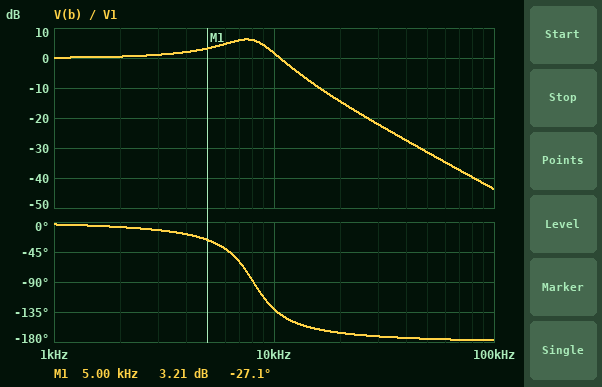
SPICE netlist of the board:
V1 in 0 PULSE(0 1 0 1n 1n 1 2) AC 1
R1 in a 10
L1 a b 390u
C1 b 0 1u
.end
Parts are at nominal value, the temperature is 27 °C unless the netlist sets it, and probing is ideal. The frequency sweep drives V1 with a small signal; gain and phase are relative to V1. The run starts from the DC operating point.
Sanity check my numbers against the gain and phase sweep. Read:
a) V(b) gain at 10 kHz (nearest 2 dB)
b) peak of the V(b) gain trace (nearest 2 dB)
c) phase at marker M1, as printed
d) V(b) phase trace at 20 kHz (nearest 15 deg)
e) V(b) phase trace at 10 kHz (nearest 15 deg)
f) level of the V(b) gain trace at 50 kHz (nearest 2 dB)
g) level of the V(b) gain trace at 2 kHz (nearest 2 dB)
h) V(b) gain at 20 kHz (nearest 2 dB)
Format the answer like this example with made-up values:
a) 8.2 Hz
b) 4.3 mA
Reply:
a) 2 dB
b) 6 dB
c) -27.1 deg
d) -165 deg
e) -135 deg
f) -32 dB
g) 0 dB
h) -14 dB
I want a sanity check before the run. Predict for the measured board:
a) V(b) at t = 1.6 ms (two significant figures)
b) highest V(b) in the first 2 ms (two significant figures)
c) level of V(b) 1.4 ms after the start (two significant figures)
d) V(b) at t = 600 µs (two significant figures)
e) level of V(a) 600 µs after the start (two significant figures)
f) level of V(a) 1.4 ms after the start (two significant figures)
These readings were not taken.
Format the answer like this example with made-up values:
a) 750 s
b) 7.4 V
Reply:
a) 1.0 V
b) 1.4 V
c) 1.0 V
d) 1.0 V
e) 1.0 V
f) 1.0 V
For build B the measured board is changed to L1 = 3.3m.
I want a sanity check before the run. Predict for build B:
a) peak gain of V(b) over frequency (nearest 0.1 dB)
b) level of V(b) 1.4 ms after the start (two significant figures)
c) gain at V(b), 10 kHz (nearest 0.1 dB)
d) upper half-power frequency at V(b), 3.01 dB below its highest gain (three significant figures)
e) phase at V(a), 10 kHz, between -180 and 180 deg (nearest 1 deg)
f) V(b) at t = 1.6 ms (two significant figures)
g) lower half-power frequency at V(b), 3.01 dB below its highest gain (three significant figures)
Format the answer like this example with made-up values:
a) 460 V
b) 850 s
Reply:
a) 15.2 dB
b) 930 mV
c) -21.6 dB
d) 2.98 kHz
e) 3 deg
f) 1.1 V
g) 2.50 kHz
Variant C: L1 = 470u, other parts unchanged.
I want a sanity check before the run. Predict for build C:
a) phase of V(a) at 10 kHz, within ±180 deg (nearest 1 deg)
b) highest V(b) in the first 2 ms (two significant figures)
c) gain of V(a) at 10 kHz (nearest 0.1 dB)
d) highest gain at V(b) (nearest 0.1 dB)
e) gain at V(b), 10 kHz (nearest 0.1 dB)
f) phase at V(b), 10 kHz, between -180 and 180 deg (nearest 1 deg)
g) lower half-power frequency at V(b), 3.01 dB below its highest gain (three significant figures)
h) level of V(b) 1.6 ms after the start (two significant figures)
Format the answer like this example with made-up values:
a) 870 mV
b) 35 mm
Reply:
a) 36 deg
b) 1.5 V
c) -1.9 dB
d) 7.0 dB
e) -0.5 dB
f) -144 deg
g) 4.90 kHz
h) 1.0 V
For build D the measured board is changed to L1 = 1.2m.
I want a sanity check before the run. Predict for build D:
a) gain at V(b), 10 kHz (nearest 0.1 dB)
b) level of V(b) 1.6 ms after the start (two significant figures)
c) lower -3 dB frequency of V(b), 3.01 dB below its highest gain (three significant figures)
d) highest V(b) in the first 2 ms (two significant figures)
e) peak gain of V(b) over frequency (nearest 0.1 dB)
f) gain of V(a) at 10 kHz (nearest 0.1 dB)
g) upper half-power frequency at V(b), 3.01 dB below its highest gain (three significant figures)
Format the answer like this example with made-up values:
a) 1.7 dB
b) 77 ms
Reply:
a) -11.6 dB
b) 1.0 V
c) 3.77 kHz
d) 1.6 V
e) 10.9 dB
f) -0.1 dB
g) 5.12 kHz
